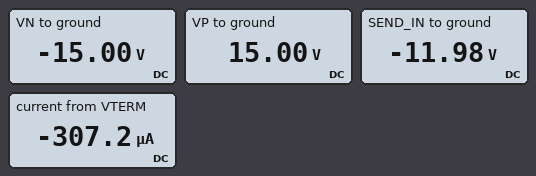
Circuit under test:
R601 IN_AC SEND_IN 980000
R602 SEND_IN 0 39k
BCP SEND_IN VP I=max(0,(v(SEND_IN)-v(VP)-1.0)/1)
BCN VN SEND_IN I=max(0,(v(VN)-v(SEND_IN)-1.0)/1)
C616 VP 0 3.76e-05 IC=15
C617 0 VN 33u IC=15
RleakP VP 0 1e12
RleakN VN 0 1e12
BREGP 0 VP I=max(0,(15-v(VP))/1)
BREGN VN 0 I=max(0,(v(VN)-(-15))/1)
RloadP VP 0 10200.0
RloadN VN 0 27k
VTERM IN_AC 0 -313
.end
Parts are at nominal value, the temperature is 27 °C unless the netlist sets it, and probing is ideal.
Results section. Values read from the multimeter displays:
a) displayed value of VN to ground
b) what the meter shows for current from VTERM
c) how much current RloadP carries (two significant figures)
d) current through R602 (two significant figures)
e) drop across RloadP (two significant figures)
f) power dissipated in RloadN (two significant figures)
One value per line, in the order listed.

-15.00 V
-307.2 µA
1.5 mA
310 µA
15 V
8.3 mW
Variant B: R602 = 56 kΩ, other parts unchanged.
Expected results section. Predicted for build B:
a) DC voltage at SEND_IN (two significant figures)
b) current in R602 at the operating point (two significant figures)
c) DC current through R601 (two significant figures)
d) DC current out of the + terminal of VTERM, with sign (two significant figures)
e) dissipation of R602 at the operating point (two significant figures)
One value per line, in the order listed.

-16 V
290 µA
300 µA
-300 µA
4.6 mW
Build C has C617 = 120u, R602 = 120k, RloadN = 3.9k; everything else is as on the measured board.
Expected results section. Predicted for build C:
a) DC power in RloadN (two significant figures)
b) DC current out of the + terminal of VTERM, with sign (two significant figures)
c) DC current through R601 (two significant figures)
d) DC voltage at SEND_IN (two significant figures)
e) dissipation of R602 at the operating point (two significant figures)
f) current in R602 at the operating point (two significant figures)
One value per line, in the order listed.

58 mW
-300 µA
300 µA
-16 V
2.1 mW
130 µA
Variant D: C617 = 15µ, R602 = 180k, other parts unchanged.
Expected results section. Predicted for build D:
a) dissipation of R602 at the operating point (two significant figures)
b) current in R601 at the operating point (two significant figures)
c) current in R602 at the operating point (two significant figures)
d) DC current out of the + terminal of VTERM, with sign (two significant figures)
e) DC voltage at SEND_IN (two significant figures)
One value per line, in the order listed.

1.4 mW
300 µA
89 µA
-300 µA
-16 V
